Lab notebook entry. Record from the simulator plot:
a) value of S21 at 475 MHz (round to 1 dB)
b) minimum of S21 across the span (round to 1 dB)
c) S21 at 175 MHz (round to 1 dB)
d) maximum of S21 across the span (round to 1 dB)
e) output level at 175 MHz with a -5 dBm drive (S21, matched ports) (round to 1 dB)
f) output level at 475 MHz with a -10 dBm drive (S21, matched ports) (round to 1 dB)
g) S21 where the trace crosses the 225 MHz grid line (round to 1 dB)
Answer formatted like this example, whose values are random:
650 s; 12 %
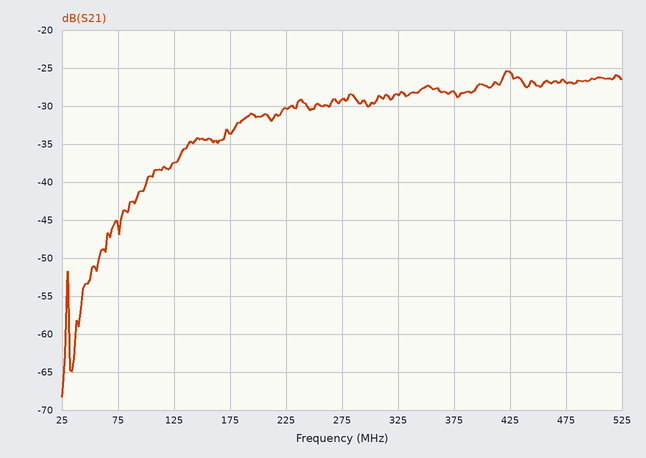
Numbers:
-27 dB; -68 dB; -34 dB; -25 dB; -39 dBm; -37 dBm; -30 dB
